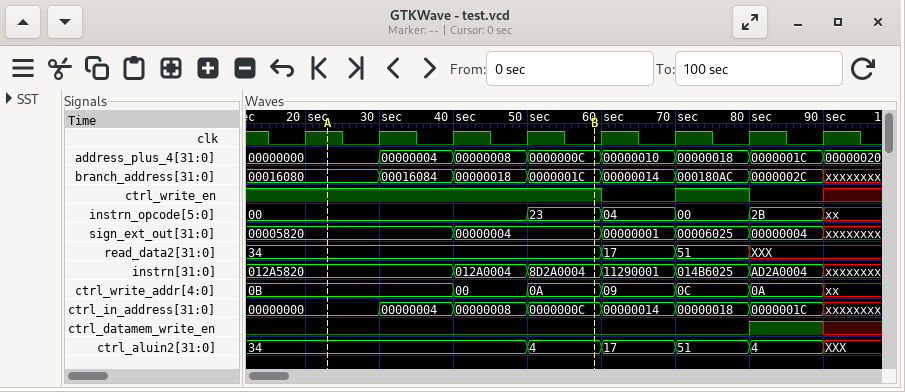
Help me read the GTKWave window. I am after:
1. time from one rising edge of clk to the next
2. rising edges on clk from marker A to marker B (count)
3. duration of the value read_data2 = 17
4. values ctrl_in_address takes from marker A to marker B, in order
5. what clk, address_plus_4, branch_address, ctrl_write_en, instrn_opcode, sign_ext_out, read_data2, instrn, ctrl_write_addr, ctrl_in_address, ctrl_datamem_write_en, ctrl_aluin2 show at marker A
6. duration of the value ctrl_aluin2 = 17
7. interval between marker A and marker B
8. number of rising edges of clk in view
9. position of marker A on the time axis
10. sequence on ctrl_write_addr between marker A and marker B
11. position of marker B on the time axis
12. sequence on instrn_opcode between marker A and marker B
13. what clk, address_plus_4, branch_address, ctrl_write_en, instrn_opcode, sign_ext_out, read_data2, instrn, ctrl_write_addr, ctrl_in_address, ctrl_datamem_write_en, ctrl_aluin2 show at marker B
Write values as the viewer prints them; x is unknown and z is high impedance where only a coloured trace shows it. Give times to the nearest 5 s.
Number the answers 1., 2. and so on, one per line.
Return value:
1. 10 s
2. 3
3. 10 s
4. 00000000, 00000004, 00000008, 0000000C
5. clk=1, address_plus_4=00000000, branch_address=00016080, ctrl_write_en=1, instrn_opcode=00, sign_ext_out=00005820, read_data2=34, instrn=012A5820, ctrl_write_addr=0B, ctrl_in_address=00000000, ctrl_datamem_write_en=0, ctrl_aluin2=34
6. 10 s
7. 35 s
8. 8
9. 25 s
10. 0B, 00, 0A
11. 60 s
12. 00, 23
13. clk=0, address_plus_4=0000000C, branch_address=0000001C, ctrl_write_en=1, instrn_opcode=23, sign_ext_out=00000004, read_data2=34, instrn=8D2A0004, ctrl_write_addr=0A, ctrl_in_address=0000000C, ctrl_datamem_write_en=0, ctrl_aluin2=4
